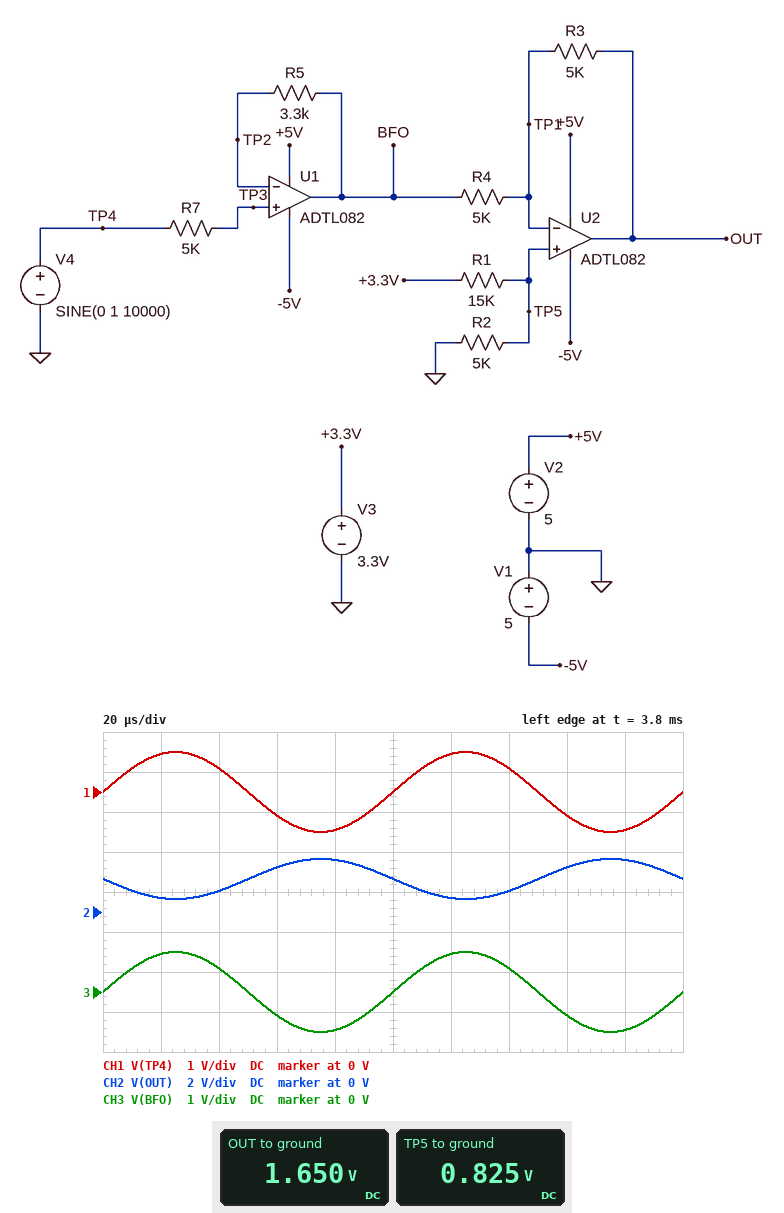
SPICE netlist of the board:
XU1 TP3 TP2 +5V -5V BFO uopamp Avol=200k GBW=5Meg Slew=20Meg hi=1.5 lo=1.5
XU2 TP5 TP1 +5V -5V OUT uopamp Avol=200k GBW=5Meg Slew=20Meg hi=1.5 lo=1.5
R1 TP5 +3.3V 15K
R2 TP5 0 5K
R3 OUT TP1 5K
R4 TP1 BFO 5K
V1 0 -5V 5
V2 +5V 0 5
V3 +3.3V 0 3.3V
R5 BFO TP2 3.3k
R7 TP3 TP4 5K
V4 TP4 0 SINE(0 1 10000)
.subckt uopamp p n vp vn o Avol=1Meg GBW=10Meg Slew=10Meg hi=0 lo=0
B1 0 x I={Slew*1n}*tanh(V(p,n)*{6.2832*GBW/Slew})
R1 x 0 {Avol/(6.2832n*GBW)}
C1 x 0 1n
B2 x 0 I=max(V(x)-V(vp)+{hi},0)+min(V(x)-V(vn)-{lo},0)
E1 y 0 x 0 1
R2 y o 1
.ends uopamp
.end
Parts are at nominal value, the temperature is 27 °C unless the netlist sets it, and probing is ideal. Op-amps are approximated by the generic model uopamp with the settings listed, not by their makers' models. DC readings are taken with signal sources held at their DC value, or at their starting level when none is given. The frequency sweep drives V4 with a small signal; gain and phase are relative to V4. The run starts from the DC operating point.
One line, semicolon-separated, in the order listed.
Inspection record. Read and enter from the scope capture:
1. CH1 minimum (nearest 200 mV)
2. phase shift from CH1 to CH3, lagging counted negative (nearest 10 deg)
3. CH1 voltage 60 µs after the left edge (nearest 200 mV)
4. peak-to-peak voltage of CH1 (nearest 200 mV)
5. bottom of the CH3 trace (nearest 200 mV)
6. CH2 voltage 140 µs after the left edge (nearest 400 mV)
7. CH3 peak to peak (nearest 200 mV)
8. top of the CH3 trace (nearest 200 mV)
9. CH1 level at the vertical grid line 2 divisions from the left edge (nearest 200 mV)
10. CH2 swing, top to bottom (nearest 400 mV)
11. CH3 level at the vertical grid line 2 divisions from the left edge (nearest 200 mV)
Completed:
-1.0 V; 0 deg; -600 mV; 2.0 V; -1.0 V; 1.2 V; 2.0 V; 1.0 V; 600 mV; 2.0 V; 600 mV
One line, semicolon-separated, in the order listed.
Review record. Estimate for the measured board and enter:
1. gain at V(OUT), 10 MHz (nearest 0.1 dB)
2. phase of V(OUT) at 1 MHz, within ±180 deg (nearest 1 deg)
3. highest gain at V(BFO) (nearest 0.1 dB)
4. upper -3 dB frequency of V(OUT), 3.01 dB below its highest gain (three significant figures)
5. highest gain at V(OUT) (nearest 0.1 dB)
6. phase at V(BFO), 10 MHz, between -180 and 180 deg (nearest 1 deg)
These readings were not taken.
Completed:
-19.3 dB; 147 deg; 0 dB; 2.09 MHz; 0 dB; -63 deg
